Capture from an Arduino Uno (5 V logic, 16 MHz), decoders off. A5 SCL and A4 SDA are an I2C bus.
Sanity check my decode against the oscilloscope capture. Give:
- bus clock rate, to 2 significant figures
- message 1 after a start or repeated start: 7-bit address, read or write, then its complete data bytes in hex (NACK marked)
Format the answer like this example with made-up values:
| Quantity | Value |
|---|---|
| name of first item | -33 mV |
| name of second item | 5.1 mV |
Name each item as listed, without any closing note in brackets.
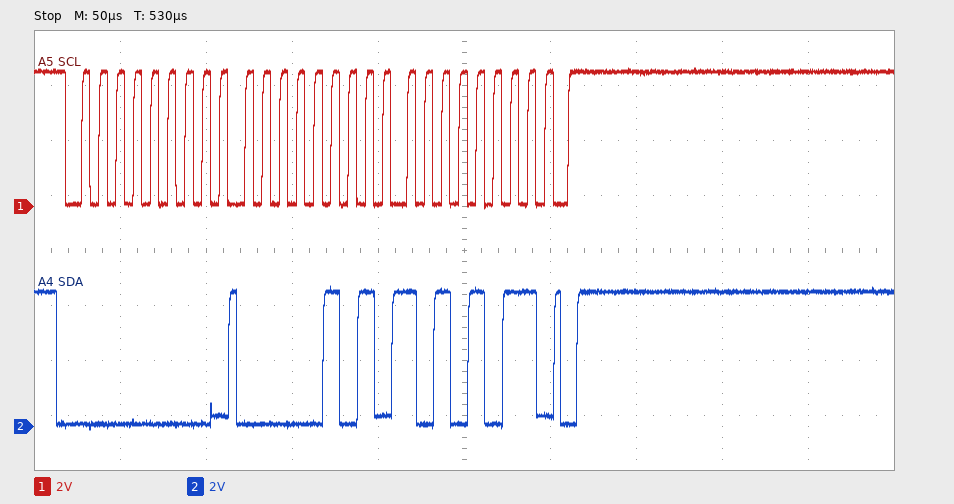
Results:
| Quantity | Value |
|---|---|
| bus clock rate, to 2 significant figures | 100 kHz |
| message 1 after a start or repeated start: 7-bit address, read or write, then its complete data bytes in hex | 0x00 write: 05 AB |
